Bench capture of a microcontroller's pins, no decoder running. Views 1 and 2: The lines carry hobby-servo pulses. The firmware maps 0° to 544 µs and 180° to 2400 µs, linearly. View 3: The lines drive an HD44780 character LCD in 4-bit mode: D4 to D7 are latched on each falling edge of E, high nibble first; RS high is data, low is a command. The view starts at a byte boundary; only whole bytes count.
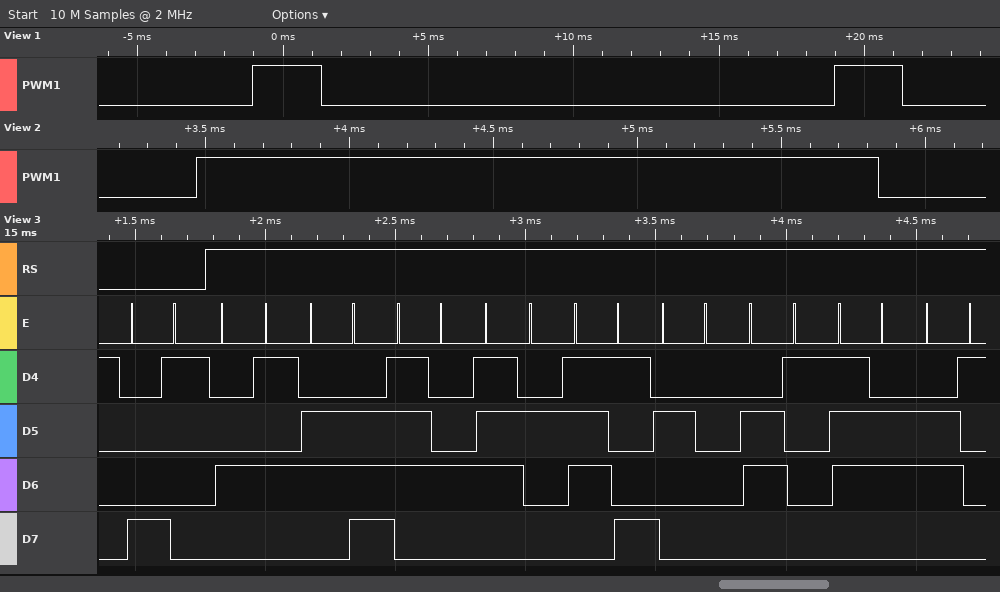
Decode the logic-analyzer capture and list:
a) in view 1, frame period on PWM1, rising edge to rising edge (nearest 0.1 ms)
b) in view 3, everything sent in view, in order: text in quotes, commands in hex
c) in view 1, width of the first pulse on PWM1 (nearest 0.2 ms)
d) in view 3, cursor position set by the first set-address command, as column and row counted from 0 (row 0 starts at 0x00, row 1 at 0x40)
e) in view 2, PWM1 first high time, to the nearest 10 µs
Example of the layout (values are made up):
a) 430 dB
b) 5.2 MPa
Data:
a) 20.0 ms
b) 0x81 "Entry ava"
c) 2.4 ms
d) column 1, row 0
e) 2370 µs
